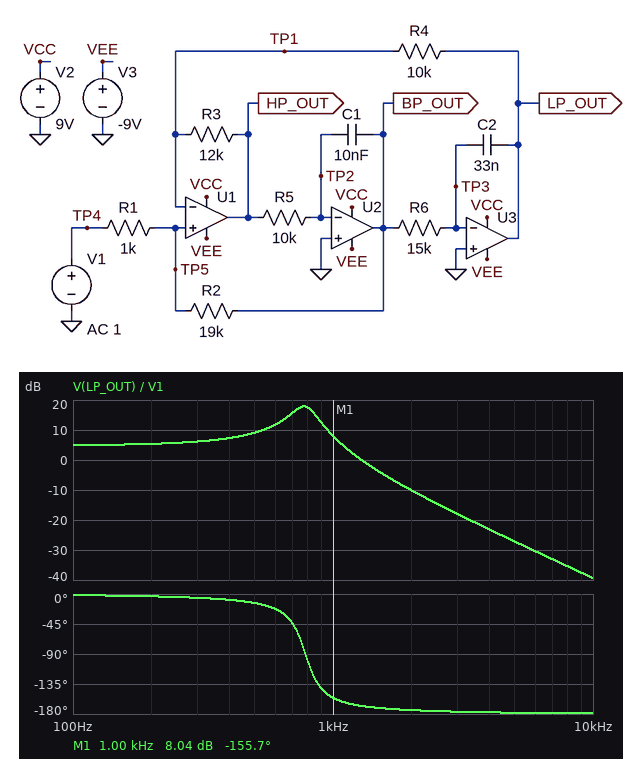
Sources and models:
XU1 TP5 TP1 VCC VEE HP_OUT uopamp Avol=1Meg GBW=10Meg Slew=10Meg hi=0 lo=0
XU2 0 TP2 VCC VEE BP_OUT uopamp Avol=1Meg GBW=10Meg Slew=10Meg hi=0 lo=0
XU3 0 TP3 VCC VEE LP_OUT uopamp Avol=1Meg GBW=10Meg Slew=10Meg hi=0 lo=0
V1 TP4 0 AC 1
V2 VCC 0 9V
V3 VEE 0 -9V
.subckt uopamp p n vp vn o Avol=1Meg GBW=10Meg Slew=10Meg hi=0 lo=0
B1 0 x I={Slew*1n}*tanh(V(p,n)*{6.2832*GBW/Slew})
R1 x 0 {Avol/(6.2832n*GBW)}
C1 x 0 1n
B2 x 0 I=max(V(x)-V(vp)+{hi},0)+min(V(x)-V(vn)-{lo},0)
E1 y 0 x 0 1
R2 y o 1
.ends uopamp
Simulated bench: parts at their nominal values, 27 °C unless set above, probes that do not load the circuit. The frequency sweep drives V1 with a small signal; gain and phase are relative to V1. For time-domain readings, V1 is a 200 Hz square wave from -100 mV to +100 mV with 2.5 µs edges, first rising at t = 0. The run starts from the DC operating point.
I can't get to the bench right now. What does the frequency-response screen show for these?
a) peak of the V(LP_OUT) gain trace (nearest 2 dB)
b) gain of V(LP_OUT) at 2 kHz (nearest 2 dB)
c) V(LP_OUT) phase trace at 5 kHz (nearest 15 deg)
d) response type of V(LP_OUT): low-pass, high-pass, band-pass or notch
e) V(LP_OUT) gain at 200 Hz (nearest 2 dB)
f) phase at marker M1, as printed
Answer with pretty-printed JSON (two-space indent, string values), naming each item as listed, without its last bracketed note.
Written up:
{
  "peak of the V(LP_OUT) gain trace": "18 dB",
  "gain of V(LP_OUT) at 2 kHz": "-10 dB",
  "V(LP_OUT) phase trace at 5 kHz": "-180 deg",
  "response type of V(LP_OUT): low-pass, high-pass, band-pass or notch": "low-pass",
  "V(LP_OUT) gain at 200 Hz": "6 dB",
  "phase at marker M1, as printed": "-155.7 deg"
}
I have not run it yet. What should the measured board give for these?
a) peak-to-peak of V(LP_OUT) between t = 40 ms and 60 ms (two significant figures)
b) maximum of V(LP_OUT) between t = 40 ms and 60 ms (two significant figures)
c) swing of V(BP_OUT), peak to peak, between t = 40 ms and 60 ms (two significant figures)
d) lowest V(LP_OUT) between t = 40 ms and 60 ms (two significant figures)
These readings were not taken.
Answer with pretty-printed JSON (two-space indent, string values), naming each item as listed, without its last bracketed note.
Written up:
{
  "peak-to-peak of V(LP_OUT) between t = 40 ms and 60 ms": "750 mV",
  "maximum of V(LP_OUT) between t = 40 ms and 60 ms": "370 mV",
  "swing of V(BP_OUT), peak to peak, between t = 40 ms and 60 ms": "1.2 V",
  "lowest V(LP_OUT) between t = 40 ms and 60 ms": "-370 mV"
}
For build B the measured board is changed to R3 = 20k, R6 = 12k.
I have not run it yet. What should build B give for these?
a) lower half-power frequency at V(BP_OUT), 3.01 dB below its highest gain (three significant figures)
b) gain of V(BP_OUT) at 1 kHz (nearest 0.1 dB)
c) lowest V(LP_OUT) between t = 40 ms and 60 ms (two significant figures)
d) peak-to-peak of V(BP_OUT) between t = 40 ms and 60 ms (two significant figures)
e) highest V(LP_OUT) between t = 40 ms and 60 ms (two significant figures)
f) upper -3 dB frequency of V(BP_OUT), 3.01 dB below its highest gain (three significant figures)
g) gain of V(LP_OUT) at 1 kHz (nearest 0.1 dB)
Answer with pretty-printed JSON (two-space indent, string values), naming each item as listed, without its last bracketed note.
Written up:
{
  "lower half-power frequency at V(BP_OUT), 3.01 dB below its highest gain": "1.02 kHz",
  "gain of V(BP_OUT) at 1 kHz": "21.8 dB",
  "lowest V(LP_OUT) between t = 40 ms and 60 ms": "-340 mV",
  "peak-to-peak of V(BP_OUT) between t = 40 ms and 60 ms": "1.3 V",
  "highest V(LP_OUT) between t = 40 ms and 60 ms": "340 mV",
  "upper -3 dB frequency of V(BP_OUT), 3.01 dB below its highest gain": "1.26 kHz",
  "gain of V(LP_OUT) at 1 kHz": "13.9 dB"
}
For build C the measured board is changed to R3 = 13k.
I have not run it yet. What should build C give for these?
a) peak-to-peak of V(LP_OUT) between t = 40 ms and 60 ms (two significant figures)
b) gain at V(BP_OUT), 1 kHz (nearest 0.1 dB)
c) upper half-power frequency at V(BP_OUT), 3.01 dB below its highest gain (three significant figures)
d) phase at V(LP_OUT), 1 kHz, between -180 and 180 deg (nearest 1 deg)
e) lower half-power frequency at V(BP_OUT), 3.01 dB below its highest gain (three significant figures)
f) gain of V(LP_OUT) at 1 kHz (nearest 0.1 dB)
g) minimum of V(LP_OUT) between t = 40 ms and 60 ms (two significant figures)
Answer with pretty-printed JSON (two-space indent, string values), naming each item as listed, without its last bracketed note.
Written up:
{
  "peak-to-peak of V(LP_OUT) between t = 40 ms and 60 ms": "720 mV",
  "gain at V(BP_OUT), 1 kHz": "19.2 dB",
  "upper half-power frequency at V(BP_OUT), 3.01 dB below its highest gain": "912 Hz",
  "phase at V(LP_OUT), 1 kHz, between -180 and 180 deg": "-151 deg",
  "lower half-power frequency at V(BP_OUT), 3.01 dB below its highest gain": "729 Hz",
  "gain of V(LP_OUT) at 1 kHz": "9.3 dB",
  "minimum of V(LP_OUT) between t = 40 ms and 60 ms": "-360 mV"
}
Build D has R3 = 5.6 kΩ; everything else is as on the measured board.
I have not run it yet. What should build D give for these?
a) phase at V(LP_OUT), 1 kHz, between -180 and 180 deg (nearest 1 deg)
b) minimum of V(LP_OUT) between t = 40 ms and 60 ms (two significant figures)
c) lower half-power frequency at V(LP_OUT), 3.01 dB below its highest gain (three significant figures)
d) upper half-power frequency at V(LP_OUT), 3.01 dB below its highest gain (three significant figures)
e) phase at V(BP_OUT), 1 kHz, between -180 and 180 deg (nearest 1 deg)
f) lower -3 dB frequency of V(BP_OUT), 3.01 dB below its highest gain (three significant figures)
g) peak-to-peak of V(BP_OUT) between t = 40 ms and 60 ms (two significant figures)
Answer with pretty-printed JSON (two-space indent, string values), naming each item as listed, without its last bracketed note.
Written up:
{
  "phase at V(LP_OUT), 1 kHz, between -180 and 180 deg": "-170 deg",
  "minimum of V(LP_OUT) between t = 40 ms and 60 ms": "-660 mV",
  "lower half-power frequency at V(LP_OUT), 3.01 dB below its highest gain": "461 Hz",
  "upper half-power frequency at V(LP_OUT), 3.01 dB below its highest gain": "587 Hz",
  "phase at V(BP_OUT), 1 kHz, between -180 and 180 deg": "100 deg",
  "lower -3 dB frequency of V(BP_OUT), 3.01 dB below its highest gain": "477 Hz",
  "peak-to-peak of V(BP_OUT) between t = 40 ms and 60 ms": "1.6 V"
}
